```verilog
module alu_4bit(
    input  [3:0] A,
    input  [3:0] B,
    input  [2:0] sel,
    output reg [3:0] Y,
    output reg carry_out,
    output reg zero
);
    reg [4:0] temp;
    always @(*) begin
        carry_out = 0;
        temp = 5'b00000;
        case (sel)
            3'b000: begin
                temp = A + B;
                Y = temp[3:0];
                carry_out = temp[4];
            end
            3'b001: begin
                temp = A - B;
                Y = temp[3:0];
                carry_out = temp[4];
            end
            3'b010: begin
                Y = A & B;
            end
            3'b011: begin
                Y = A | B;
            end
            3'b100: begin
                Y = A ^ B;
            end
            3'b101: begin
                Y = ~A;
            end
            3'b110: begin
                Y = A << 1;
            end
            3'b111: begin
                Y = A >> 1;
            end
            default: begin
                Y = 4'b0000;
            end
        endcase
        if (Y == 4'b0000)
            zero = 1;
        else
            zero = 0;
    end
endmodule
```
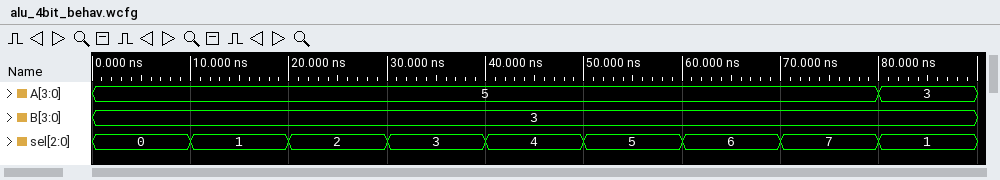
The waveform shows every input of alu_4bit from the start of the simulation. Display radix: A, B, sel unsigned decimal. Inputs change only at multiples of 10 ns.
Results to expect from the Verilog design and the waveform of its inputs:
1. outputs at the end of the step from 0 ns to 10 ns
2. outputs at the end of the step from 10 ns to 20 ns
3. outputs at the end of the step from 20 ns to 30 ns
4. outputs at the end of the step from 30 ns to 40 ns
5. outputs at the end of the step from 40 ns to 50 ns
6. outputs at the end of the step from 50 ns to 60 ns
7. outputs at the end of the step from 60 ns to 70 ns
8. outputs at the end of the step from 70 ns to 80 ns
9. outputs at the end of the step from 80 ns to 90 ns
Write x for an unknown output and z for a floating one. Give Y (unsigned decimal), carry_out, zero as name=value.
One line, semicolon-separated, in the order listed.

Y=8, carry_out=0, zero=0; Y=2, carry_out=0, zero=0; Y=1, carry_out=0, zero=0; Y=7, carry_out=0, zero=0; Y=6, carry_out=0, zero=0; Y=10, carry_out=0, zero=0; Y=10, carry_out=0, zero=0; Y=2, carry_out=0, zero=0; Y=0, carry_out=0, zero=1
